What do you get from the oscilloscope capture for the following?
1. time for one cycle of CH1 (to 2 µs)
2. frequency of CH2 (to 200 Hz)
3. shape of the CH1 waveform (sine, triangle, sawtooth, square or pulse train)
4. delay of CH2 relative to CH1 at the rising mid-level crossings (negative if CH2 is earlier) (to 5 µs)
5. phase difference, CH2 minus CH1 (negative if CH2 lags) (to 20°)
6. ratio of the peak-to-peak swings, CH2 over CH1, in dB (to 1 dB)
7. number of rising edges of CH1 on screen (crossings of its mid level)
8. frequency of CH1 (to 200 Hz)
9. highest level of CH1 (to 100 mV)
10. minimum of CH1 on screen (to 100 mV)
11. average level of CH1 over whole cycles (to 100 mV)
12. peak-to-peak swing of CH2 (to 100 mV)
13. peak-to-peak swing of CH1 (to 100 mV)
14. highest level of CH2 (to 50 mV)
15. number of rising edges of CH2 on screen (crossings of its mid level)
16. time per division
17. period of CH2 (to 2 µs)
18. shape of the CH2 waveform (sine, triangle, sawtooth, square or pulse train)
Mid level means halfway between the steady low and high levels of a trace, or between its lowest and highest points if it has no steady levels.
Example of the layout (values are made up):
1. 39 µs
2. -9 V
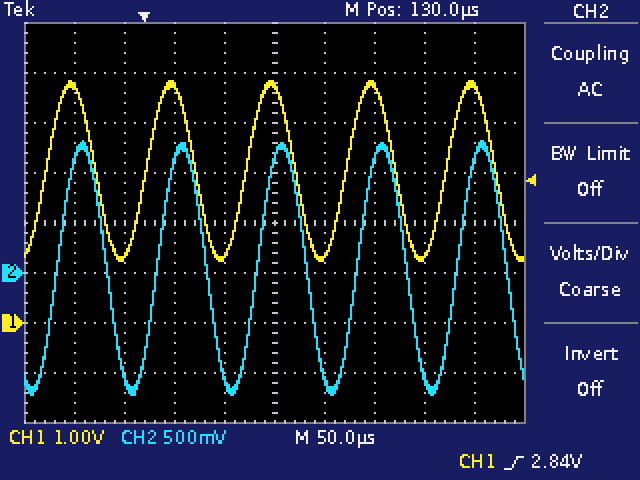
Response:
1. 100 µs
2. 10.0 kHz
3. sine
4. +10 µs
5. -40°
6. -3 dB
7. 5
8. 10.0 kHz
9. 4.8 V
10. 1.2 V
11. 3.0 V
12. 2.50 V
13. 3.6 V
14. 1.30 V
15. 5
16. 50 µs
17. 100 µs
18. sine
